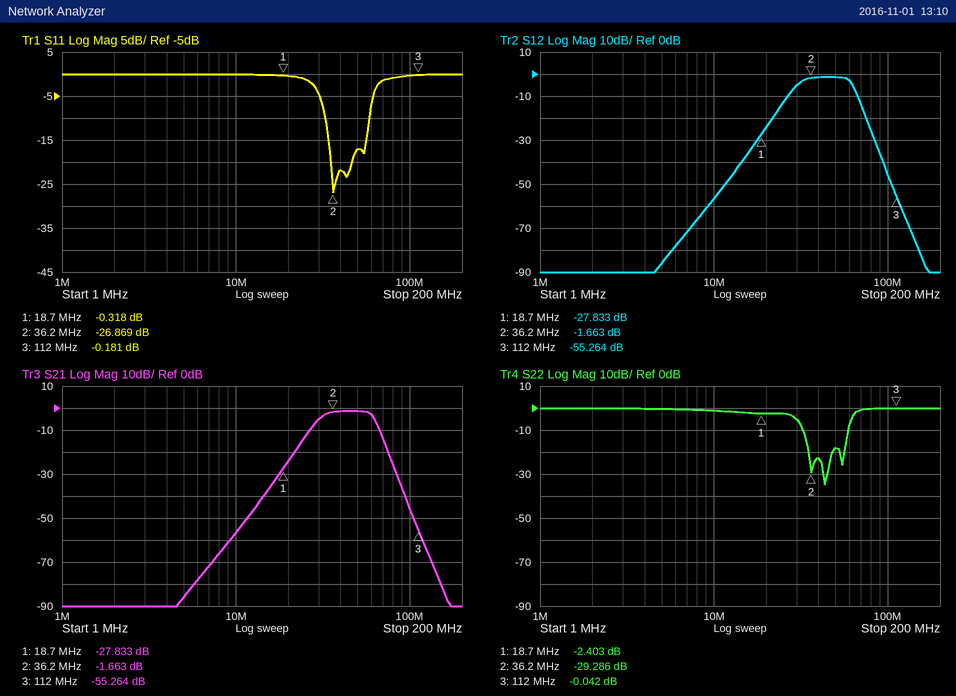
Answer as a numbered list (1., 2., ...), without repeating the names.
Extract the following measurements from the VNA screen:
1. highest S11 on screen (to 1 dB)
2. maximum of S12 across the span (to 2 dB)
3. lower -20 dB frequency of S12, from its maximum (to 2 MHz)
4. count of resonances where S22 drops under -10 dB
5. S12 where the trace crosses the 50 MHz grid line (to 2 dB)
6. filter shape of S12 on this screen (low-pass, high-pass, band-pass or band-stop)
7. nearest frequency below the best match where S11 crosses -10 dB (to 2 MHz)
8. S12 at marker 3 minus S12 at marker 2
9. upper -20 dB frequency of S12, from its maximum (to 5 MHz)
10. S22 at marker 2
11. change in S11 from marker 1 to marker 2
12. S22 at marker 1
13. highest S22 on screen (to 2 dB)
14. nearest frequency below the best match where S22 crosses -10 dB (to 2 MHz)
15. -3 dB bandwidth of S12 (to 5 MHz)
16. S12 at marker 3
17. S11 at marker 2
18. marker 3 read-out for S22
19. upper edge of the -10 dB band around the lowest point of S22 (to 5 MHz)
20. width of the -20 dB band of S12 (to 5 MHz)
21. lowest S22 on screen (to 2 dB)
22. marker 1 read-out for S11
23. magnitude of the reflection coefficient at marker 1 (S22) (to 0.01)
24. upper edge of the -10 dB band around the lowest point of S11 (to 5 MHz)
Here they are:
1. 0 dB
2. -2 dB
3. 22 MHz
4. 3
5. -2 dB
6. band-pass
7. 32 MHz
8. -53.601 dB
9. 75 MHz
10. -29.286 dB
11. -26.551 dB
12. -2.403 dB
13. 0 dB
14. 32 MHz
15. 30 MHz
16. -55.264 dB
17. -26.869 dB
18. -0.042 dB
19. 60 MHz
20. 55 MHz
21. -34 dB
22. -0.318 dB
23. 0.76
24. 60 MHz
